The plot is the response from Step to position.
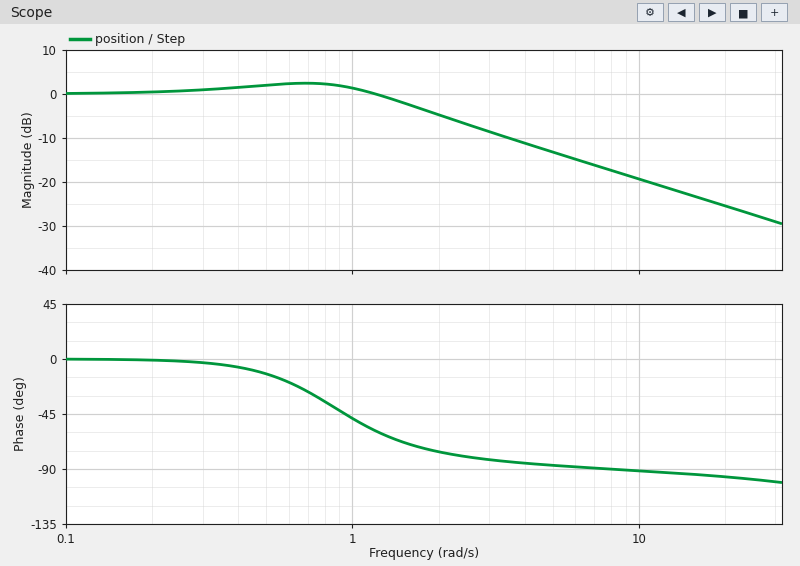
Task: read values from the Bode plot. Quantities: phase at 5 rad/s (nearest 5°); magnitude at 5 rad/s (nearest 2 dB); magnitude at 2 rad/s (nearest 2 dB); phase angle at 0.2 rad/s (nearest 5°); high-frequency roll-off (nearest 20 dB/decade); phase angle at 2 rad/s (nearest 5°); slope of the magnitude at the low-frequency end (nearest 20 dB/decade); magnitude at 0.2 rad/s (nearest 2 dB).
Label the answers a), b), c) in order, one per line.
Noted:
a) -85°
b) -14 dB
c) -4 dB
d) 0°
e) -20 dB/decade
f) -75°
g) 0 dB/decade
h) 0 dB
